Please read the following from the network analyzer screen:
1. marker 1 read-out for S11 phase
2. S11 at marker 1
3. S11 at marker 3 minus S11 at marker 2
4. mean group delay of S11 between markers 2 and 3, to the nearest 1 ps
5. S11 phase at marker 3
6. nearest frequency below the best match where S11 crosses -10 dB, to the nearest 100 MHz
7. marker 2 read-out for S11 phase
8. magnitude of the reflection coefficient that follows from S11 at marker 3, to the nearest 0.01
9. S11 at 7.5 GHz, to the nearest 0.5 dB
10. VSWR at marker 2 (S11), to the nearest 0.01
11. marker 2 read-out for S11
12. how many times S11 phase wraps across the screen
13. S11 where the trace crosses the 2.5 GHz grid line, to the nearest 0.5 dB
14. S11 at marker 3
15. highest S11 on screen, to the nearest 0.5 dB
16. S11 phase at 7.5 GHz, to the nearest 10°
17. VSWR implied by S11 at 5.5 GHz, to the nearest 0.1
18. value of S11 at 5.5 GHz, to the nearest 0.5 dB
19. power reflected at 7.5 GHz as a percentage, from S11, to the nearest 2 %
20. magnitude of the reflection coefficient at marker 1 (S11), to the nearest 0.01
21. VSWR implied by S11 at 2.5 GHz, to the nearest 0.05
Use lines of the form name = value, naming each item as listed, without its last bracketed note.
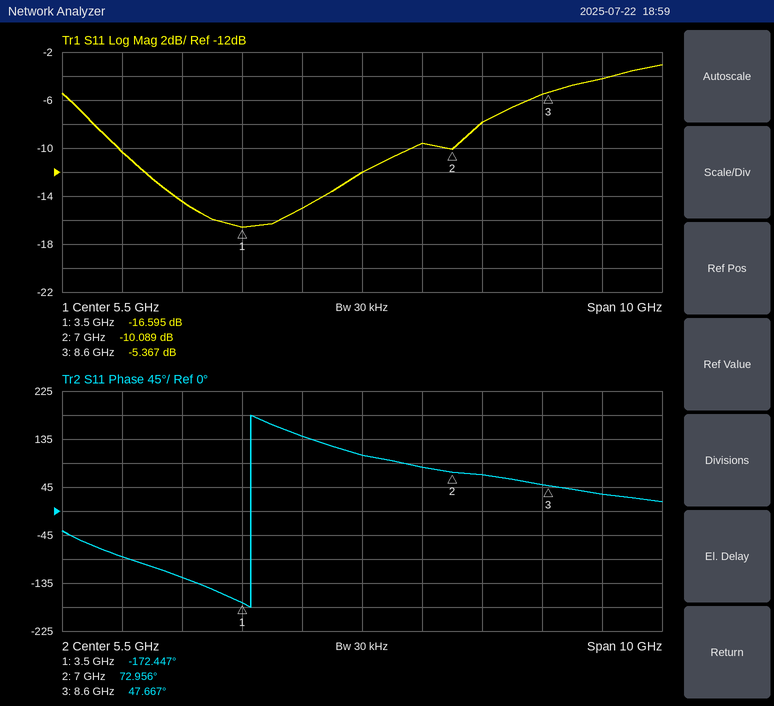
marker 1 read-out for S11 phase = -172.447°
S11 at marker 1 = -16.595 dB
S11 at marker 3 minus S11 at marker 2 = 4.722 dB
mean group delay of S11 between markers 2 and 3, to the nearest 1 ps = 44 ps
S11 phase at marker 3 = 47.667°
nearest frequency below the best match where S11 crosses -10 dB, to the nearest 100 MHz = 1.4 GHz
marker 2 read-out for S11 phase = 72.956°
magnitude of the reflection coefficient that follows from S11 at marker 3, to the nearest 0.01 = 0.54
S11 at 7.5 GHz, to the nearest 0.5 dB = -8.0 dB
VSWR at marker 2 (S11), to the nearest 0.01 = 1.91
marker 2 read-out for S11 = -10.089 dB
how many times S11 phase wraps across the screen = 1
S11 where the trace crosses the 2.5 GHz grid line, to the nearest 0.5 dB = -14.5 dB
S11 at marker 3 = -5.367 dB
highest S11 on screen, to the nearest 0.5 dB = -3.0 dB
S11 phase at 7.5 GHz, to the nearest 10° = 70°
VSWR implied by S11 at 5.5 GHz, to the nearest 0.1 = 1.7
value of S11 at 5.5 GHz, to the nearest 0.5 dB = -12.0 dB
power reflected at 7.5 GHz as a percentage, from S11, to the nearest 2 % = 16 %
magnitude of the reflection coefficient at marker 1 (S11), to the nearest 0.01 = 0.15
VSWR implied by S11 at 2.5 GHz, to the nearest 0.05 = 1.45
